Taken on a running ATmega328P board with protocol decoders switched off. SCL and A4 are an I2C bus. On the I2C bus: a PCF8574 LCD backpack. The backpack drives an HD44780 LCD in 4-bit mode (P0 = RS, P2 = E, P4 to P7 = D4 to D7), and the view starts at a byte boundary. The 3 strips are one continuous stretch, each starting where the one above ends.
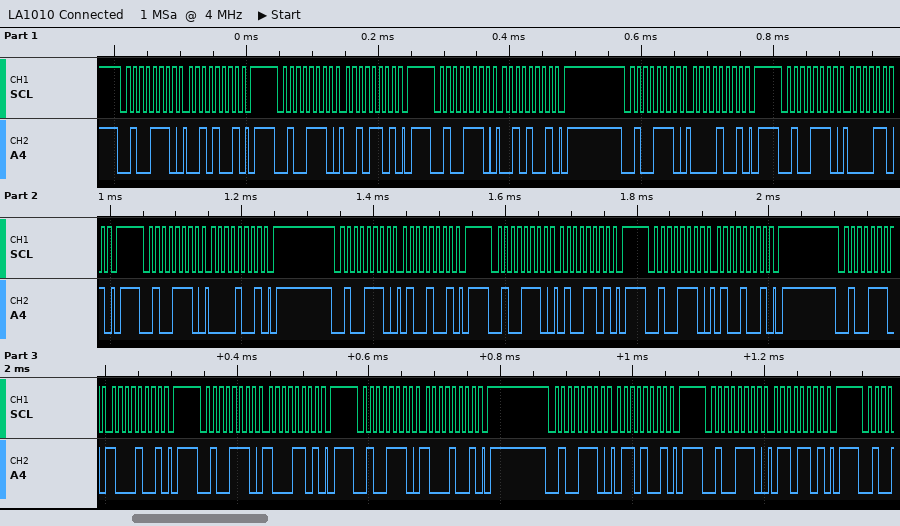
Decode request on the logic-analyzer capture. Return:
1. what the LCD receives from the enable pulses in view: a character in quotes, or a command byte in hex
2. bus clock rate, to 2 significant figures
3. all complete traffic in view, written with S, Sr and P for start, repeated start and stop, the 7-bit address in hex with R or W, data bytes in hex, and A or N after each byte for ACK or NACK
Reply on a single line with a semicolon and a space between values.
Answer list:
' ' 'H'; 100 kHz; S 27W A 29 A P S 27W A 2D A P S 27W A 29 A P S 27W A 09 A P S 27W A 0D A P S 27W A 09 A P S 27W A 49 A P S 27W A 4D A P S 27W A 49 A P S 27W A 89 A P S 27W A 8D A P S 27W A 89 A P S 27W A 69 A P S 27W A 6D A P
